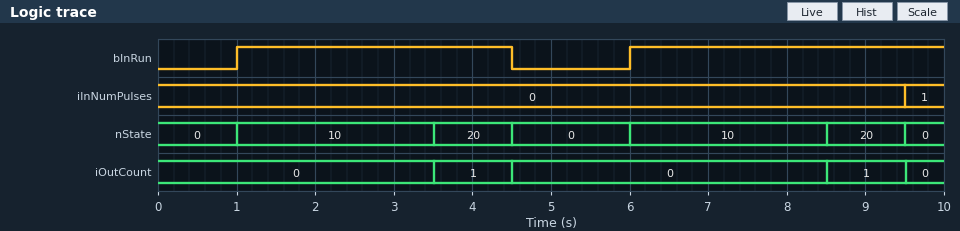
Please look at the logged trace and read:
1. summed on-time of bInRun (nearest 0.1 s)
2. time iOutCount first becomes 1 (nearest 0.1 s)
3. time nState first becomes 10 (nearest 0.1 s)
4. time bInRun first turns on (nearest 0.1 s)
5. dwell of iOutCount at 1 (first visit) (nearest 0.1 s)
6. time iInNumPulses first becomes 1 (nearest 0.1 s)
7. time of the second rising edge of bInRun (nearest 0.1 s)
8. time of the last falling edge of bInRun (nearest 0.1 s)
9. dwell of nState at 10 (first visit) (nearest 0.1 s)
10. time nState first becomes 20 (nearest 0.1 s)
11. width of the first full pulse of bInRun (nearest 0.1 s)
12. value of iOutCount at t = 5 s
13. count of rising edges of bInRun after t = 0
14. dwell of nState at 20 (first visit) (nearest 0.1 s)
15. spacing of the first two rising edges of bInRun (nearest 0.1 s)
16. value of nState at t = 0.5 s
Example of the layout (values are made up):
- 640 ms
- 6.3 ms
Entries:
- 7.5 s
- 3.5 s
- 1.0 s
- 1.0 s
- 1.0 s
- 9.5 s
- 6.0 s
- 4.5 s
- 2.5 s
- 3.5 s
- 3.5 s
- 0
- 2
- 1.0 s
- 5.0 s
- 0
